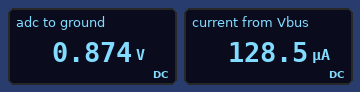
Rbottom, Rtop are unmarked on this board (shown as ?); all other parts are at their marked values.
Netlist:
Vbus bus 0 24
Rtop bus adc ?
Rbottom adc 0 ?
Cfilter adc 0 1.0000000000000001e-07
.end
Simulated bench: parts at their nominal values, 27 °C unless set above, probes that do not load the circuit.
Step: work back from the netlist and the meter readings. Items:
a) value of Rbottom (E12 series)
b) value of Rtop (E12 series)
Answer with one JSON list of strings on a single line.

["6.8 kΩ", "180 kΩ"]
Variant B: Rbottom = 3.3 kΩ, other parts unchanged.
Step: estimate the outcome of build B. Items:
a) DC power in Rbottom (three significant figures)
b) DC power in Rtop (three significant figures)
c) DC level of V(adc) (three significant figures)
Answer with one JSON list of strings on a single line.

["56.6 µW", "3.09 mW", "432 mV"]
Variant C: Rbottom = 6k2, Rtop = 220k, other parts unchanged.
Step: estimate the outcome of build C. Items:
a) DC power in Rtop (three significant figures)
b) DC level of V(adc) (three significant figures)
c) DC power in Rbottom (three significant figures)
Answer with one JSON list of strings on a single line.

["2.48 mW", "658 mV", "69.8 µW"]
